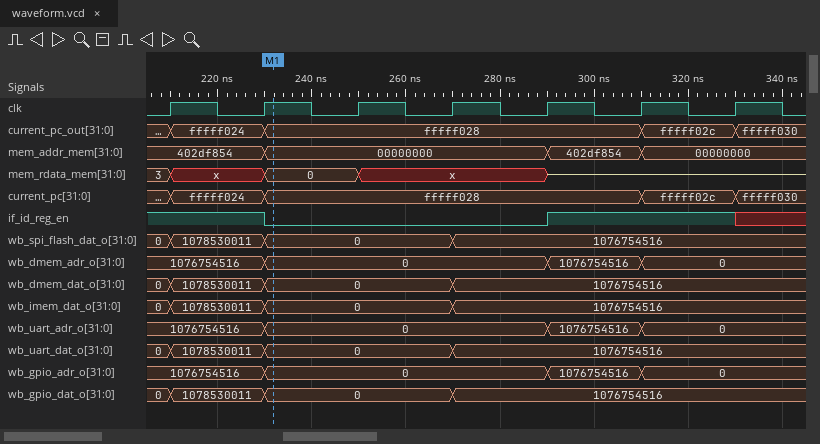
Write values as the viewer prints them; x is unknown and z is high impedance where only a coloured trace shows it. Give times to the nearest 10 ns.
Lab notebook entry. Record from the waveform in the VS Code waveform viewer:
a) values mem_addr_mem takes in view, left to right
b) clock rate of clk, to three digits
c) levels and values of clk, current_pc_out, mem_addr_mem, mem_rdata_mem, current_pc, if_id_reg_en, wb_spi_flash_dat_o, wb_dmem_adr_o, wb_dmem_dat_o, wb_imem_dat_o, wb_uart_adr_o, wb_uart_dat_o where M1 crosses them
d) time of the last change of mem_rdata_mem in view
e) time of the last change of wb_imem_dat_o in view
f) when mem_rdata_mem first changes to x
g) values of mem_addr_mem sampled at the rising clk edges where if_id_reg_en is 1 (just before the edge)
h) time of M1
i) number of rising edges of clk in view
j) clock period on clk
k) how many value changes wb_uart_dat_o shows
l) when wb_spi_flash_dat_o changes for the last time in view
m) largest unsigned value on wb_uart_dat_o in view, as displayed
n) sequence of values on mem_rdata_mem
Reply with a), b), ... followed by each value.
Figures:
a) 402df854, 00000000, 402df854, 00000000
b) 50.0 MHz
c) clk=1, current_pc_out=fffff028, mem_addr_mem=00000000, mem_rdata_mem=0, current_pc=fffff028, if_id_reg_en=0, wb_spi_flash_dat_o=0, wb_dmem_adr_o=0, wb_dmem_dat_o=0, wb_imem_dat_o=0, wb_uart_adr_o=0, wb_uart_dat_o=0
d) 290 ns
e) 270 ns
f) 210 ns
g) 402df854, 402df854, 402df854, 00000000
h) 230 ns
i) 7
j) 20 ns
k) 3
l) 270 ns
m) 1078530011
n) 3, x, 0, x, z
